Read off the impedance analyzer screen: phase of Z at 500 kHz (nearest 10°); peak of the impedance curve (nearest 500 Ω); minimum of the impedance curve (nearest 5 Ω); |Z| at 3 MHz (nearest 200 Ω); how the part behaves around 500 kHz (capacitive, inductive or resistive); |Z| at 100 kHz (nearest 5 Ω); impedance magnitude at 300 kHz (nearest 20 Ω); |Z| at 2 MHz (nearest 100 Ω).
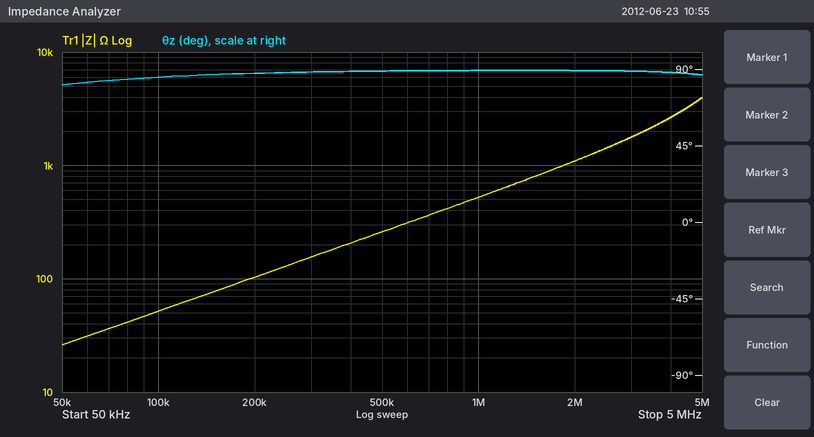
90°
4.0 kΩ
25 Ω
1.8 kΩ
inductive
50 Ω
160 Ω
1.1 kΩ
